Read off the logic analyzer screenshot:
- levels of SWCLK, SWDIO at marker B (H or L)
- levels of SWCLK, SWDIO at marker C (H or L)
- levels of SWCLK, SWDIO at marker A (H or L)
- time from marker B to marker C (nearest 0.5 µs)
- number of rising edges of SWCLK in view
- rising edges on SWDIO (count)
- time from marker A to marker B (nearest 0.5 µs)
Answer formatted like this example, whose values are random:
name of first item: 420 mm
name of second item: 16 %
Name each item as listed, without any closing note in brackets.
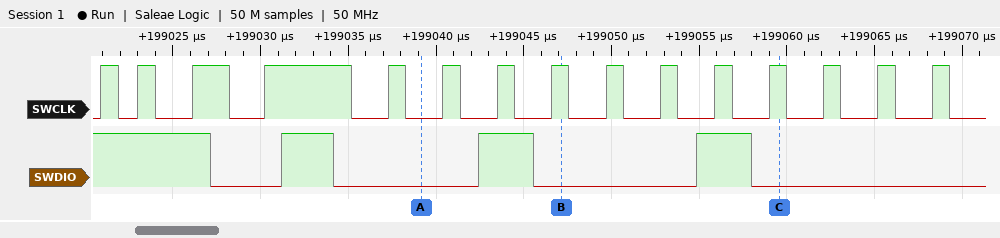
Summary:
levels of SWCLK, SWDIO at marker B: SWCLK=H, SWDIO=L
levels of SWCLK, SWDIO at marker C: SWCLK=H, SWDIO=L
levels of SWCLK, SWDIO at marker A: SWCLK=L, SWDIO=L
time from marker B to marker C: 12.5 µs
number of rising edges of SWCLK in view: 15
rising edges on SWDIO: 3
time from marker A to marker B: 8 µs
